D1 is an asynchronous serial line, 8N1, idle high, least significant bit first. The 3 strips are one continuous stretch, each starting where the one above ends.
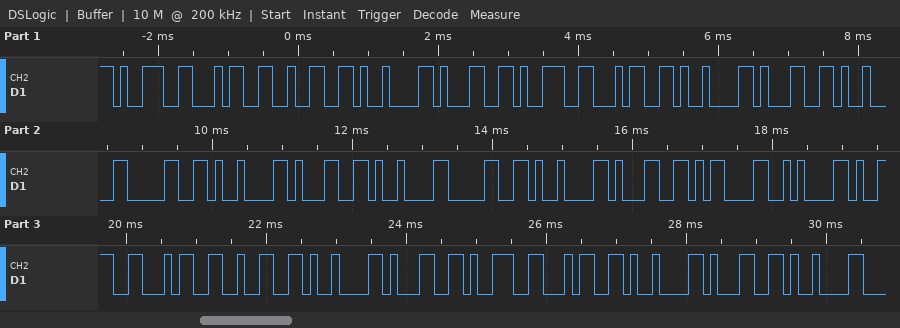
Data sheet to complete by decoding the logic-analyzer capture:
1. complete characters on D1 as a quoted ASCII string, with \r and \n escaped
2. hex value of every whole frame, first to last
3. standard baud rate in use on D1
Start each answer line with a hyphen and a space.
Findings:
- "942\t194\t1\t0\t1\t0\t1\r\n942\t194\t1\t"
- 0x39 0x34 0x32 0x09 0x31 0x39 0x34 0x09 0x31 0x09 0x30 0x09 0x31 0x09 0x30 0x09 0x31 0x0D 0x0A 0x39 0x34 0x32 0x09 0x31 0x39 0x34 0x09 0x31 0x09
- 9600 baud
